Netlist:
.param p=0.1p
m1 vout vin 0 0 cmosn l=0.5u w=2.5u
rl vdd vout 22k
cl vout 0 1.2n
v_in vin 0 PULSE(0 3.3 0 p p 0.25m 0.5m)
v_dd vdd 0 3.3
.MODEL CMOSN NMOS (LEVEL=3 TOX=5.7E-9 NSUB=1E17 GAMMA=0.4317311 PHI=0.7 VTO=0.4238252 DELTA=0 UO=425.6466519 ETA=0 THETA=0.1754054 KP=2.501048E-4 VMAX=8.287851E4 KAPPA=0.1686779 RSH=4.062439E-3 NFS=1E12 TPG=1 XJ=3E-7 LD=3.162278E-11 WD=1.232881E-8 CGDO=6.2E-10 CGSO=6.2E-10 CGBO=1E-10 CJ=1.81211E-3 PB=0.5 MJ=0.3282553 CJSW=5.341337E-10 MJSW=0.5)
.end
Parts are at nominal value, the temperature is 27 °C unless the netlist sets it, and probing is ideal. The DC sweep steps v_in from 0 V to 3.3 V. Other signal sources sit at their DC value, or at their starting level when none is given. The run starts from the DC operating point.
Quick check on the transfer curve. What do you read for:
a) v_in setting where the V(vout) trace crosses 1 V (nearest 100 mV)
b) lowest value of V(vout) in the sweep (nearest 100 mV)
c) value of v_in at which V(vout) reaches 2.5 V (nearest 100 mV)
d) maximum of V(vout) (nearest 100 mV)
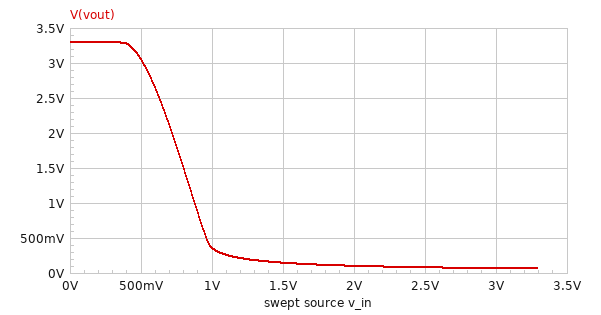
900 mV
100 mV
600 mV
3.3 V
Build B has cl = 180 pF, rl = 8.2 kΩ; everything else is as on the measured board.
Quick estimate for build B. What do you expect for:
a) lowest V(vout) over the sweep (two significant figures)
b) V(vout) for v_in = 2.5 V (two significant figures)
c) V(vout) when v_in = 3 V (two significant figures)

180 mV
240 mV
200 mV
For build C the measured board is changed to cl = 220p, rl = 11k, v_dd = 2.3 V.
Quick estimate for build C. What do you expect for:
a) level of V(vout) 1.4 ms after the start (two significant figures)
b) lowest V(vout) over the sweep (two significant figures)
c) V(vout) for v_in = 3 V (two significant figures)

2.3 V
90 mV
98 mV
